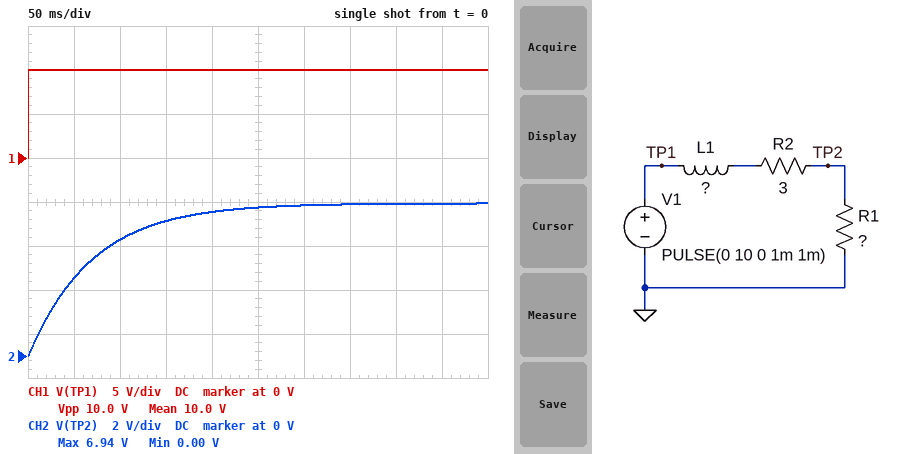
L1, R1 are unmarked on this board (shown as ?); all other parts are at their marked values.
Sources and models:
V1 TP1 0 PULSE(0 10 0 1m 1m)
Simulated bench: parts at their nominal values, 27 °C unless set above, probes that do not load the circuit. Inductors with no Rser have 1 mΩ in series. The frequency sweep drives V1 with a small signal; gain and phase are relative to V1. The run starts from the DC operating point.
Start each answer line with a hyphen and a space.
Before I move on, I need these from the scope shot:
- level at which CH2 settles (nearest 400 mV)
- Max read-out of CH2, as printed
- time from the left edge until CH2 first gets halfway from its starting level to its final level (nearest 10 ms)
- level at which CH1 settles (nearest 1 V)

- 6.8 V
- 6.94 V
- 50 ms
- 10 V
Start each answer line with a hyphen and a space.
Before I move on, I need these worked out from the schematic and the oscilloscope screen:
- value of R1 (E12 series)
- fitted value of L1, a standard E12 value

- 6.8 Ω
- 680 mH
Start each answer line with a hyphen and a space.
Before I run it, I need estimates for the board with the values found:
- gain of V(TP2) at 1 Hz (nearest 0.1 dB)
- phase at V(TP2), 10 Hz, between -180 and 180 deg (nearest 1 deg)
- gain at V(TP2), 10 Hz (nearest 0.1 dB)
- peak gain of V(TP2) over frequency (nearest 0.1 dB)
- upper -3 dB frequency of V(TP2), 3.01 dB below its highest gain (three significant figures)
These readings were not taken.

- -3.9 dB
- -77 deg
- -16.2 dB
- -3.2 dB
- 2.29 Hz
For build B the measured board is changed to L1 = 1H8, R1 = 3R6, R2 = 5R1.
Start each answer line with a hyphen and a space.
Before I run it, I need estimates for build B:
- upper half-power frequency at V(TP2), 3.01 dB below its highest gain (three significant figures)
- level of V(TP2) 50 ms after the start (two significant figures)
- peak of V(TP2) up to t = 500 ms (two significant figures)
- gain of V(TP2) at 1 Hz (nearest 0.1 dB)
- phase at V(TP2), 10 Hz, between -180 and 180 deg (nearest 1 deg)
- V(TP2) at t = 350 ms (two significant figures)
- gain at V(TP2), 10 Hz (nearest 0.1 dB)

- 769 mHz
- 880 mV
- 3.8 V
- -12.0 dB
- -86 deg
- 3.4 V
- -30.0 dB
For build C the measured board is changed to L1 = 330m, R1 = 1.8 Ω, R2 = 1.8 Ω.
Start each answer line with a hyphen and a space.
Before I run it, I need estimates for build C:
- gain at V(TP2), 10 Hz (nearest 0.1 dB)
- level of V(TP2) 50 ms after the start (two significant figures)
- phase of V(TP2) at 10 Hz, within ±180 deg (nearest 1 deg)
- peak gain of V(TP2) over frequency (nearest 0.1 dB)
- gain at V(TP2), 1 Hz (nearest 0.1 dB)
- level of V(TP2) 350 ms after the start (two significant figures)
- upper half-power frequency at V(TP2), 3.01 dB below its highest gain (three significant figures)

- -21.4 dB
- 2.1 V
- -80 deg
- -6.0 dB
- -7.3 dB
- 4.9 V
- 1.74 Hz
